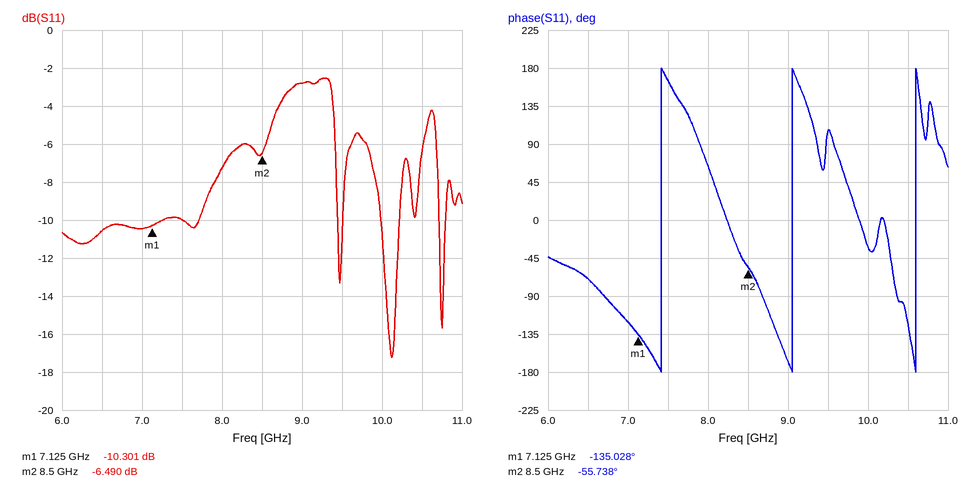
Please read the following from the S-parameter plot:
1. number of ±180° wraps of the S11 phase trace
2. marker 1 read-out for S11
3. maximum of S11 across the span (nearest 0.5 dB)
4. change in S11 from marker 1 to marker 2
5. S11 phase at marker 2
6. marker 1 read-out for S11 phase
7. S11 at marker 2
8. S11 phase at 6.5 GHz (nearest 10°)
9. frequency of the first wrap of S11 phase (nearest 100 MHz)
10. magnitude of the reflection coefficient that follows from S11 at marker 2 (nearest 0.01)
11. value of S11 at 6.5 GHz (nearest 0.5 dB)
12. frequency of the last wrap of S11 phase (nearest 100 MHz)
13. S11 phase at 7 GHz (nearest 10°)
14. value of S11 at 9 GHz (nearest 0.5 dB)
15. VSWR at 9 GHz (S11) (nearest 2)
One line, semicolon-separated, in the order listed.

3; -10.301 dB; -2.5 dB; 3.811 dB; -55.738°; -135.028°; -6.490 dB; -70°; 7.4 GHz; 0.47; -10.5 dB; 10.6 GHz; -120°; -3.0 dB; 6
